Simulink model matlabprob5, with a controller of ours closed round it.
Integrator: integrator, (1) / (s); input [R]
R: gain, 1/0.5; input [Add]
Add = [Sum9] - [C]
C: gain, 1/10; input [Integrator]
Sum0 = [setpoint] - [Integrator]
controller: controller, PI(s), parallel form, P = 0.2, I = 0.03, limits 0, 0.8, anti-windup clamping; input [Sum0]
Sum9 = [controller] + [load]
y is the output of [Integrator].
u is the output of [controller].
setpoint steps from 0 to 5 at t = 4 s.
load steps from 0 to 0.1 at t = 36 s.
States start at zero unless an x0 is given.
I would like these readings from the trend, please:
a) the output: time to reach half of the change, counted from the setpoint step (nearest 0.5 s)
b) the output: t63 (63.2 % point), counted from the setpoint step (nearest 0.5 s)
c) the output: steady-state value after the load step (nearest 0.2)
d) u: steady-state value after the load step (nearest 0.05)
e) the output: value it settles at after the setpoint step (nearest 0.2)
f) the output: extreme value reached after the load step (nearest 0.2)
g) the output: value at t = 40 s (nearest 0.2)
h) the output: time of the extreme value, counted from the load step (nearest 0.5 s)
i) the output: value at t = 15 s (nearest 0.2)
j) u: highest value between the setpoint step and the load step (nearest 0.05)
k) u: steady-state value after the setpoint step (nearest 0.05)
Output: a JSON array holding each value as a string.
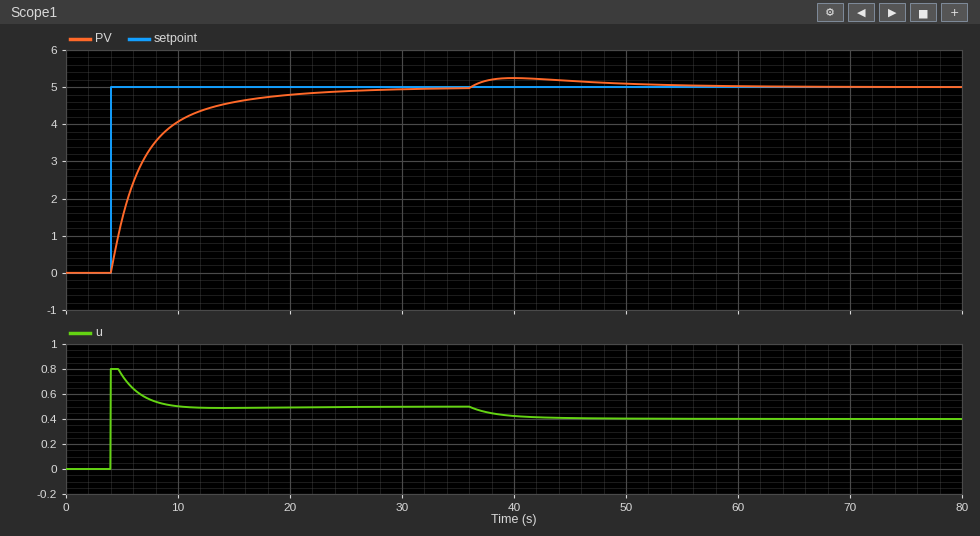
["2.0 s", "3.0 s", "5.0", "0.40", "5.0", "5.2", "5.2", "4.0 s", "4.6", "0.80", "0.50"]
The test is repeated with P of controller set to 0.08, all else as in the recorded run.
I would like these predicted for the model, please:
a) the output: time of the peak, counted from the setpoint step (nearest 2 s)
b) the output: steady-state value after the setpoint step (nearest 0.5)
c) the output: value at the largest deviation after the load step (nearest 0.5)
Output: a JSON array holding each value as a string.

["14 s", "5.0", "5.5"]
